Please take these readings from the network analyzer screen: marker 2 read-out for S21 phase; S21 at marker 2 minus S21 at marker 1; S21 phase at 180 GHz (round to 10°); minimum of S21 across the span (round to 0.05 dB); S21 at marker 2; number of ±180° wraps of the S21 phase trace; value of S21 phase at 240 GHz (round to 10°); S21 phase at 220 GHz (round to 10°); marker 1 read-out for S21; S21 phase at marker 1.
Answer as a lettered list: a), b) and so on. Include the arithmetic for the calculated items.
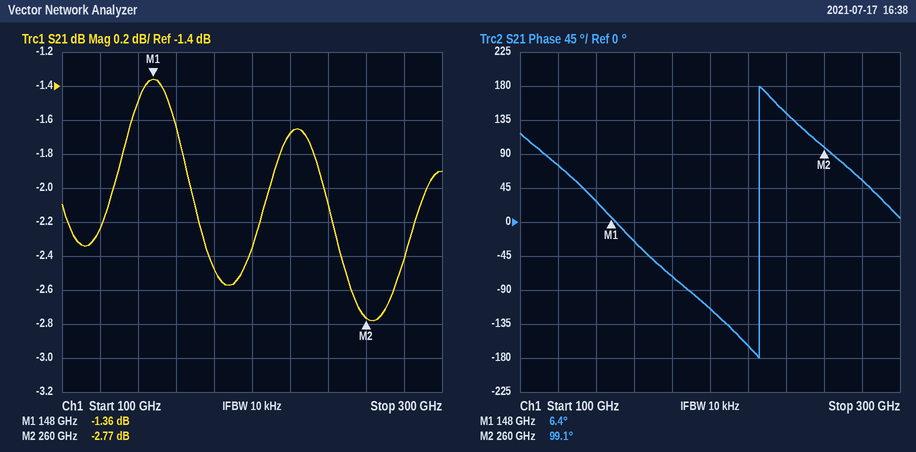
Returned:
a) 99.1°
b) -2.77 − (-1.36) = -1.41 dB
c) -70°
d) -2.80 dB
e) -2.77 dB
f) 1
g) 140°
h) -160°
i) -1.36 dB
j) 6.4°
